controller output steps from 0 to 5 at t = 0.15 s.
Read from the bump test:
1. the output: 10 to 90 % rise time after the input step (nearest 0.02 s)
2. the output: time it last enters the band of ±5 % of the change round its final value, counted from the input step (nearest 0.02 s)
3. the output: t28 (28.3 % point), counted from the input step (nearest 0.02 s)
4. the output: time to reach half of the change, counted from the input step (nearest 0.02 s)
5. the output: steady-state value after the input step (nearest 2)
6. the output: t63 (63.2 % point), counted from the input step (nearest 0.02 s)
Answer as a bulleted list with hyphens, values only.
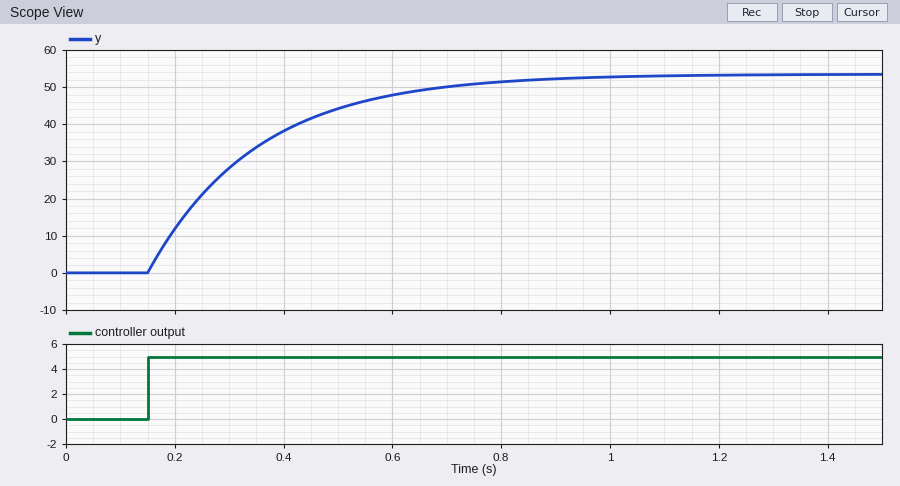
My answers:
- 0.44 s
- 0.60 s
- 0.06 s
- 0.14 s
- 54
- 0.20 s
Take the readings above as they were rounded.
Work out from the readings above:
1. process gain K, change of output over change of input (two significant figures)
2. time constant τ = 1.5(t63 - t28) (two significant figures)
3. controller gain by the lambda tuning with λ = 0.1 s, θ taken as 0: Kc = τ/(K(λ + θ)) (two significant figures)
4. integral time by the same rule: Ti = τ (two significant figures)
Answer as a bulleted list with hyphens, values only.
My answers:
- 11
- 0.21 s
- 0.19
- 0.21 s
